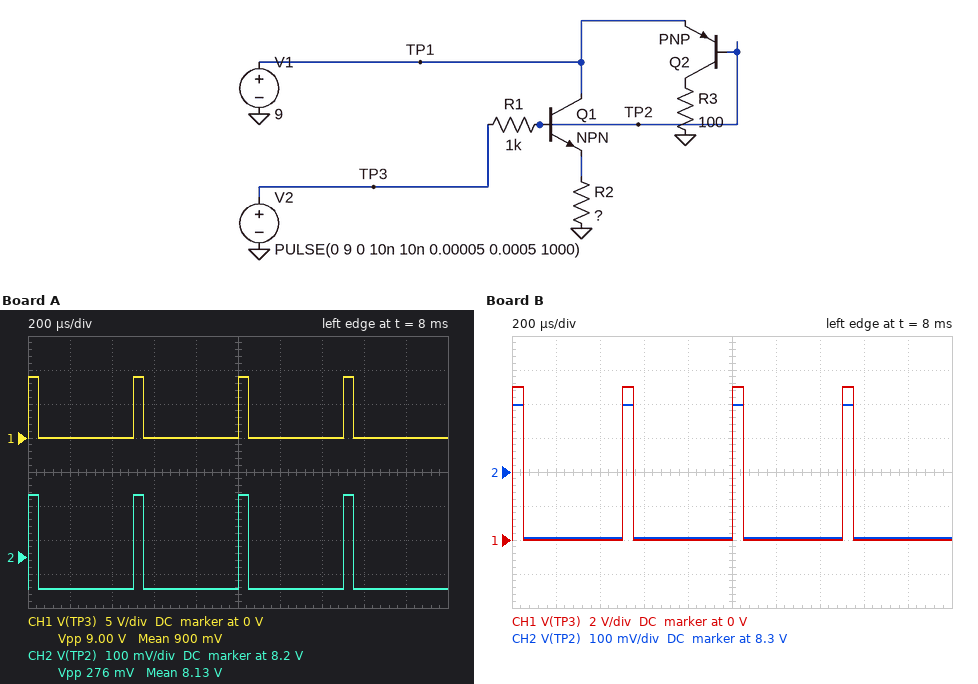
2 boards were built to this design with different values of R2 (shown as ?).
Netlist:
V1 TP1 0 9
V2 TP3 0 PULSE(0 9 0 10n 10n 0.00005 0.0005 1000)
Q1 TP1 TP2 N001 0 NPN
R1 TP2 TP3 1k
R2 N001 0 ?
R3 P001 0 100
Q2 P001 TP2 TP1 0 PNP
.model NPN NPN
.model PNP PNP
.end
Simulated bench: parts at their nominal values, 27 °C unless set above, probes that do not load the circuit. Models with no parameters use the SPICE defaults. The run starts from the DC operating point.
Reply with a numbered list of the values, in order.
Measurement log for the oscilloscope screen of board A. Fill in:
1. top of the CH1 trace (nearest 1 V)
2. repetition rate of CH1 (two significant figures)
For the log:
1. 9 V
2. 2.0 kHz
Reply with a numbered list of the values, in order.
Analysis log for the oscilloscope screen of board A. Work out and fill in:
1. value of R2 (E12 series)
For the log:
1. 120 Ω
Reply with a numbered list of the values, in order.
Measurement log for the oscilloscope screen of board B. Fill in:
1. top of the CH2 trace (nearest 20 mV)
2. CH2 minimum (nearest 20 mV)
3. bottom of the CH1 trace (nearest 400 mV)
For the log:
1. 8.50 V
2. 8.10 V
3. 0 V
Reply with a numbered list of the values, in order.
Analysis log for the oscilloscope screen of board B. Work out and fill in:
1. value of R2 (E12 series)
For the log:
1. 150 Ω
